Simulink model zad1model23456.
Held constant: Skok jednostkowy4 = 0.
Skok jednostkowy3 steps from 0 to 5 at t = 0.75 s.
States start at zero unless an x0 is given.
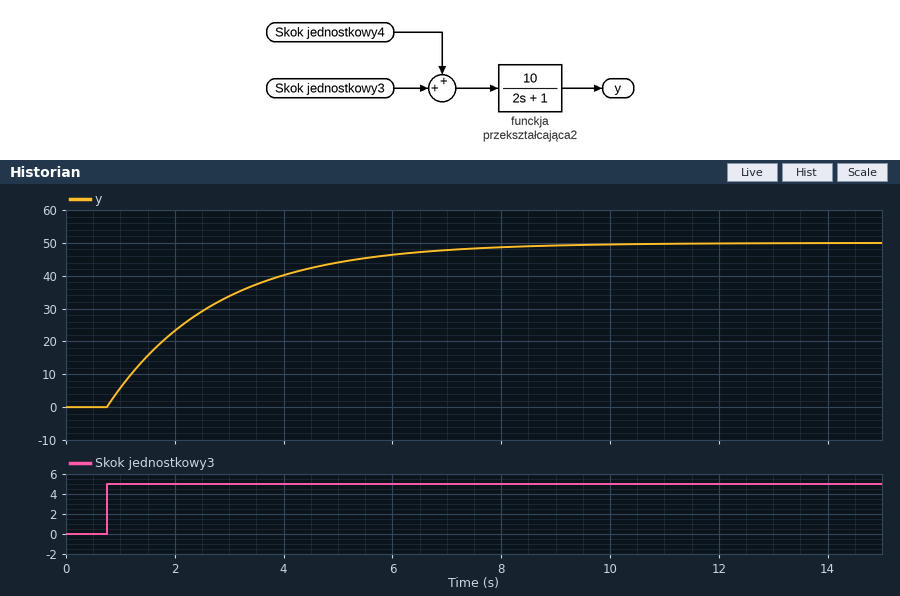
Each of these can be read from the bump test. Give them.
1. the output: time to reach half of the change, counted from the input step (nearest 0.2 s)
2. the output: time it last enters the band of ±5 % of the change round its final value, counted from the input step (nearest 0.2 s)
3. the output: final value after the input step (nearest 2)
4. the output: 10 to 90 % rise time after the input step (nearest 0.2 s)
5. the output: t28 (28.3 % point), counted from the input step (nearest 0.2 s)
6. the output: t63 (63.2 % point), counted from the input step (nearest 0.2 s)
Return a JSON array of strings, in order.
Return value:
["1.4 s", "6.0 s", "50", "4.4 s", "0.6 s", "2.0 s"]
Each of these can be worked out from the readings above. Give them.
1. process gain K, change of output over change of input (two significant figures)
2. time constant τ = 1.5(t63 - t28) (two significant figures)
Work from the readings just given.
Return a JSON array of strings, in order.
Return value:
["10", "2.1 s"]
